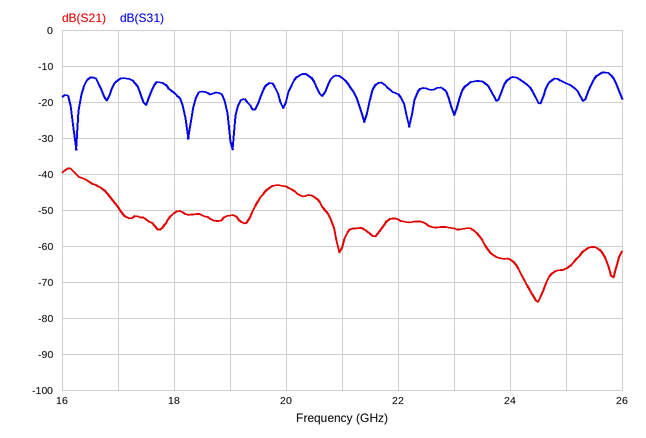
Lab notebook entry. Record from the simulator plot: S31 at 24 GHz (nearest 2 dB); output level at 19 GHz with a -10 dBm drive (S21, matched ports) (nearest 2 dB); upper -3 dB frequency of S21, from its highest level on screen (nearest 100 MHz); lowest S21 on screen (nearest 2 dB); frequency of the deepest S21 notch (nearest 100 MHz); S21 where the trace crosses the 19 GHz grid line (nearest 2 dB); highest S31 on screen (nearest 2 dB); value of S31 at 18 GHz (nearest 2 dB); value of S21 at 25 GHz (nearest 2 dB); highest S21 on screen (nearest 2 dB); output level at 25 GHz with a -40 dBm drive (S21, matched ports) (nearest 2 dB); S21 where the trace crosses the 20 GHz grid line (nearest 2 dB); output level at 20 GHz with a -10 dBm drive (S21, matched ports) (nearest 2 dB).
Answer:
-14 dB
-62 dBm
16.4 GHz
-76 dB
24.5 GHz
-52 dB
-12 dB
-18 dB
-66 dB
-38 dB
-106 dBm
-44 dB
-54 dBm
